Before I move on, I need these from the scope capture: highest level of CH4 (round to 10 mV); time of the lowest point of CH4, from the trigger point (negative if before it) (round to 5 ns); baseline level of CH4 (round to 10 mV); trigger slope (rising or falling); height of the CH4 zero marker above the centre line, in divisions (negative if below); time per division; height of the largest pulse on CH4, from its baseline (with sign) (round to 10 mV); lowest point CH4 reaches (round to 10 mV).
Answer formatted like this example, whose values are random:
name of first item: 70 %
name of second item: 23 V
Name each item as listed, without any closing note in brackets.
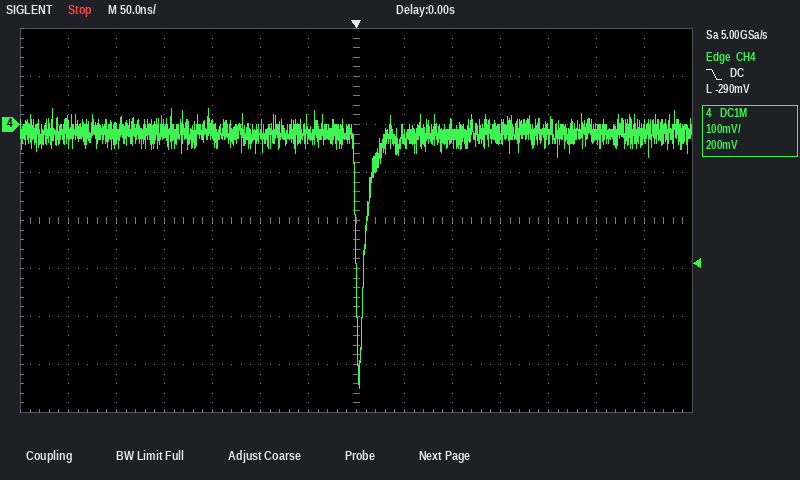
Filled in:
highest level of CH4: 30 mV
time of the lowest point of CH4, from the trigger point (negative if before it): +5 ns
baseline level of CH4: -20 mV
trigger slope: falling
height of the CH4 zero marker above the centre line, in divisions: +2.0 div
time per division: 50 ns
height of the largest pulse on CH4, from its baseline (with sign): -530 mV
lowest point CH4 reaches: -550 mV
